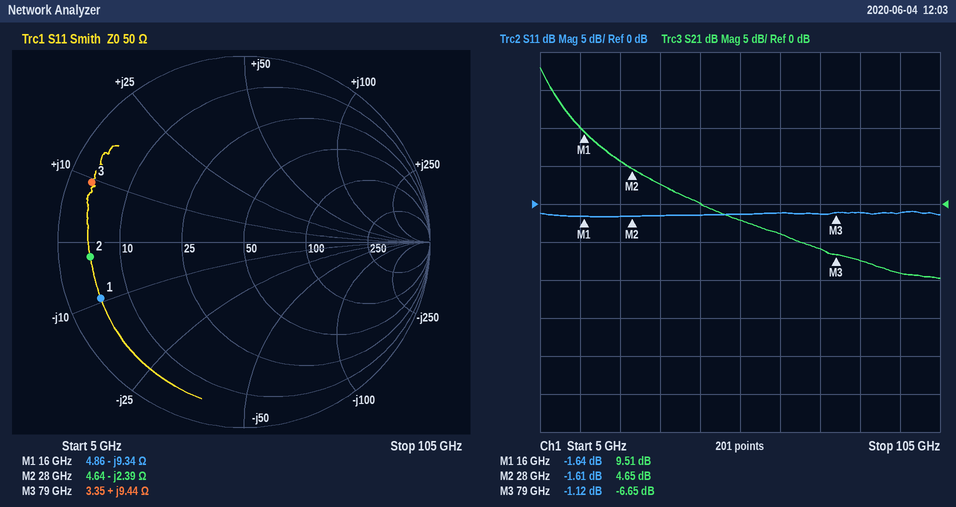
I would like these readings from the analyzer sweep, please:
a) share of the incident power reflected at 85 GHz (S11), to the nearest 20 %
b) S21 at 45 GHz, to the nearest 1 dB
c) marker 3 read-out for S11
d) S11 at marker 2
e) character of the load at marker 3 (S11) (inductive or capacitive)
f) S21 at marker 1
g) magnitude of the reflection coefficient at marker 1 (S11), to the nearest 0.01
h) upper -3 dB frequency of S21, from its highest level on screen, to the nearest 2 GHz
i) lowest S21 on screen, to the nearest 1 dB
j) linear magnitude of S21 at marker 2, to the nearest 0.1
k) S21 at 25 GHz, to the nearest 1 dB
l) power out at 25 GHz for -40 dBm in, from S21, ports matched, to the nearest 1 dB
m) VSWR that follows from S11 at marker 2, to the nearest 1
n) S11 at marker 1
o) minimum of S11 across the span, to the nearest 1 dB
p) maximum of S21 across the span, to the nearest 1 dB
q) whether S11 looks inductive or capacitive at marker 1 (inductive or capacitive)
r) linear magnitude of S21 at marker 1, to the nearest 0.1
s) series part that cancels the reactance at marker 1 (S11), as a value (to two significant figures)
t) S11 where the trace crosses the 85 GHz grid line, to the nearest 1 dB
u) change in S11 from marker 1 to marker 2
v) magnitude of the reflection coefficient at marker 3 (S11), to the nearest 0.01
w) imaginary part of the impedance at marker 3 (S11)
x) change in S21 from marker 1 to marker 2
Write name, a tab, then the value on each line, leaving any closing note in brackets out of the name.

share of the incident power reflected at 85 GHz (S11), to the nearest 20 %	80 %
S21 at 45 GHz, to the nearest 1 dB	0 dB
marker 3 read-out for S11	-1.12 dB
S11 at marker 2	-1.61 dB
character of the load at marker 3 (S11)	inductive
S21 at marker 1	9.51 dB
magnitude of the reflection coefficient at marker 1 (S11), to the nearest 0.01	0.83
upper -3 dB frequency of S21, from its highest level on screen, to the nearest 2 GHz	8 GHz
lowest S21 on screen, to the nearest 1 dB	-10 dB
linear magnitude of S21 at marker 2, to the nearest 0.1	1.7
S21 at 25 GHz, to the nearest 1 dB	6 dB
power out at 25 GHz for -40 dBm in, from S21, ports matched, to the nearest 1 dB	-34 dBm
VSWR that follows from S11 at marker 2, to the nearest 1	11
S11 at marker 1	-1.64 dB
minimum of S11 across the span, to the nearest 1 dB	-2 dB
maximum of S21 across the span, to the nearest 1 dB	18 dB
whether S11 looks inductive or capacitive at marker 1	capacitive
linear magnitude of S21 at marker 1, to the nearest 0.1	3.0
series part that cancels the reactance at marker 1 (S11), as a value	93 pH
S11 where the trace crosses the 85 GHz grid line, to the nearest 1 dB	-1 dB
change in S11 from marker 1 to marker 2	0.03 dB
magnitude of the reflection coefficient at marker 3 (S11), to the nearest 0.01	0.88
imaginary part of the impedance at marker 3	+9.44 Ω
change in S21 from marker 1 to marker 2	-4.86 dB
